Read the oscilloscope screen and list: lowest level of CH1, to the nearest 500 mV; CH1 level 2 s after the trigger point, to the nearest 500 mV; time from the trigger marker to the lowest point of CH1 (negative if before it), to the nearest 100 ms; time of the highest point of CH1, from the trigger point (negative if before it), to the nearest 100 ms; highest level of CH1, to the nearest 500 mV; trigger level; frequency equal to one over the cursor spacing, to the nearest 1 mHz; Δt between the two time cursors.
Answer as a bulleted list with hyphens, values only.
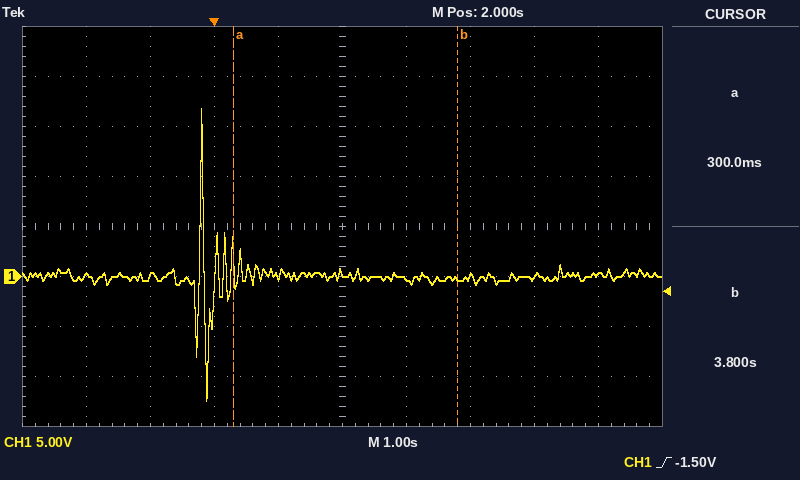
- -12.5 V
- 500 mV
- -100 ms
- -200 ms
- 17.0 V
- -1.50 V
- 286 mHz
- 3.5 s
